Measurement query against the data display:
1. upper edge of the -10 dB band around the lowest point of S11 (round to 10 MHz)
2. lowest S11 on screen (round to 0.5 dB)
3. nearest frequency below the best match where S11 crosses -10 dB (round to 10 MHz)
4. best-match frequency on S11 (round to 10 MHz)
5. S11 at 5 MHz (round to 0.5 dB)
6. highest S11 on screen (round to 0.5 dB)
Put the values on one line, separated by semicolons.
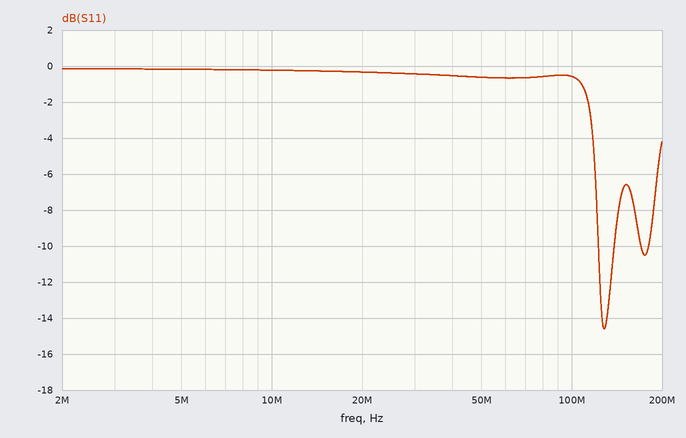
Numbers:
140 MHz; -14.5 dB; 120 MHz; 130 MHz; 0.0 dB; 0.0 dB
